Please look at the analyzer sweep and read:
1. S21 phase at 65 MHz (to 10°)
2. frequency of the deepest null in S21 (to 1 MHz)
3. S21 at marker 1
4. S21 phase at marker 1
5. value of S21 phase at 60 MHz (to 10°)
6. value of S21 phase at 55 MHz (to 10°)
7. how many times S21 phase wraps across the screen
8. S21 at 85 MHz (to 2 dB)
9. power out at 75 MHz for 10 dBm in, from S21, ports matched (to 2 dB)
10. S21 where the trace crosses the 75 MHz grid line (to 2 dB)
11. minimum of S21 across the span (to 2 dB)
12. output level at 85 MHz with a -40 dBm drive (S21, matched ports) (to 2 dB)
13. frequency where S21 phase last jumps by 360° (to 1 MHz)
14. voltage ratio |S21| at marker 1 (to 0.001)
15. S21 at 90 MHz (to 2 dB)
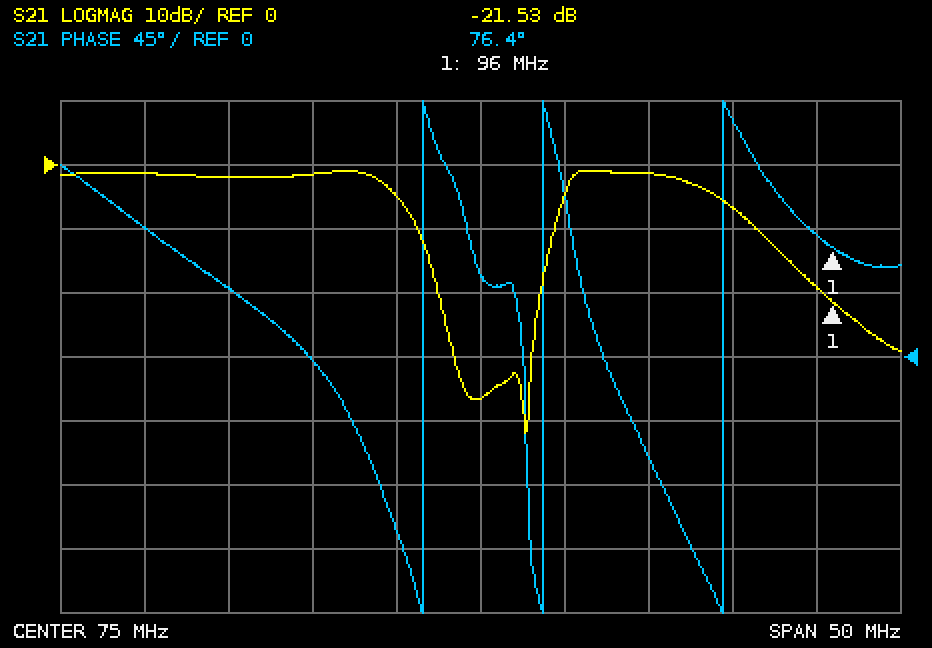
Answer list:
0°
78 MHz
-21.53 dB
76.4°
50°
90°
3
-2 dB
-26 dBm
-36 dB
-42 dB
-42 dBm
89 MHz
0.084
-6 dB
